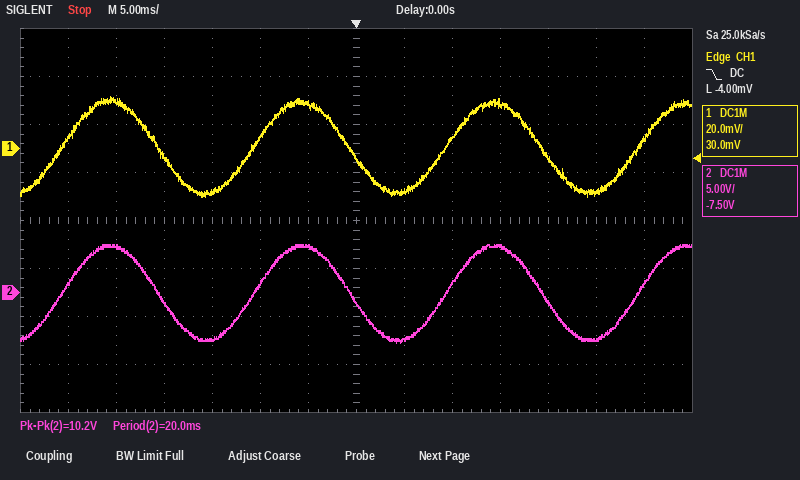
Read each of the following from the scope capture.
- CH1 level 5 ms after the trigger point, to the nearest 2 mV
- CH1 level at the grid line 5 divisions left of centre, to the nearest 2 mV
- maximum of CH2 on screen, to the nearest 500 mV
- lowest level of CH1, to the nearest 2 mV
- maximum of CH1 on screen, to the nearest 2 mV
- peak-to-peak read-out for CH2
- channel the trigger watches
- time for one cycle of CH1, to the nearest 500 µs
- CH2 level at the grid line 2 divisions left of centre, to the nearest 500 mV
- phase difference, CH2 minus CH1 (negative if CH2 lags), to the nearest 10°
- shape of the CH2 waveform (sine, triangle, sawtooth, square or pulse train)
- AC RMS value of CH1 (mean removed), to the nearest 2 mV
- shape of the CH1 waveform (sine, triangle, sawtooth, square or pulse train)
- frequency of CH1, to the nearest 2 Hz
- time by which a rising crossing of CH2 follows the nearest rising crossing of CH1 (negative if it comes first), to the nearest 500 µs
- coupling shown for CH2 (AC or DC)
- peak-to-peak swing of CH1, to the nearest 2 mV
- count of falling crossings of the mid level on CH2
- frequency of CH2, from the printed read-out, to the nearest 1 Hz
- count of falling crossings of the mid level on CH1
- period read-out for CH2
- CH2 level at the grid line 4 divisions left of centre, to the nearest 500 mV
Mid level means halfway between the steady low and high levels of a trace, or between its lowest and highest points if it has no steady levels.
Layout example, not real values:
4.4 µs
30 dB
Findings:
-18 mV
20 mV
5.0 V
-20 mV
22 mV
10.2 V
CH1
20.0 ms
1.0 V
0°
sine
14 mV
sine
50 Hz
0.0 ms
DC
42 mV
3
50 Hz
3
20.0 ms
-1.0 V
